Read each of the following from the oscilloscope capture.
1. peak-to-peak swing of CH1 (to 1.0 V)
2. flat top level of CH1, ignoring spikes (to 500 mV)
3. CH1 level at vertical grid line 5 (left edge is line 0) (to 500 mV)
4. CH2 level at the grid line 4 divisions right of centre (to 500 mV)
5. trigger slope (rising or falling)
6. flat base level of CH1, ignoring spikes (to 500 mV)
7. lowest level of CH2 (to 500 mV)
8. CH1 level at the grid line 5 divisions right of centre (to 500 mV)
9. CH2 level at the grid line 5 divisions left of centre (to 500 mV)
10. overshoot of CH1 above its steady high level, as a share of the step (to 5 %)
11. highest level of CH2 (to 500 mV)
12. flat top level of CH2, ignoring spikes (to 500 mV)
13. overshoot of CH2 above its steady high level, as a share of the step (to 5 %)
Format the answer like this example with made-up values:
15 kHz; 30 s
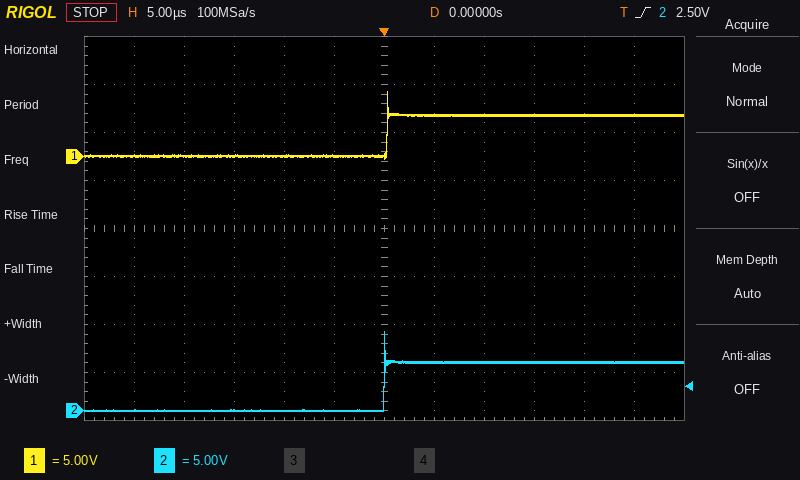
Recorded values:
7.0 V; 4.5 V; 0.0 V; 5.0 V; rising; 0.0 V; 0.0 V; 4.5 V; 0.0 V; 55 %; 8.5 V; 5.0 V; 65 %
